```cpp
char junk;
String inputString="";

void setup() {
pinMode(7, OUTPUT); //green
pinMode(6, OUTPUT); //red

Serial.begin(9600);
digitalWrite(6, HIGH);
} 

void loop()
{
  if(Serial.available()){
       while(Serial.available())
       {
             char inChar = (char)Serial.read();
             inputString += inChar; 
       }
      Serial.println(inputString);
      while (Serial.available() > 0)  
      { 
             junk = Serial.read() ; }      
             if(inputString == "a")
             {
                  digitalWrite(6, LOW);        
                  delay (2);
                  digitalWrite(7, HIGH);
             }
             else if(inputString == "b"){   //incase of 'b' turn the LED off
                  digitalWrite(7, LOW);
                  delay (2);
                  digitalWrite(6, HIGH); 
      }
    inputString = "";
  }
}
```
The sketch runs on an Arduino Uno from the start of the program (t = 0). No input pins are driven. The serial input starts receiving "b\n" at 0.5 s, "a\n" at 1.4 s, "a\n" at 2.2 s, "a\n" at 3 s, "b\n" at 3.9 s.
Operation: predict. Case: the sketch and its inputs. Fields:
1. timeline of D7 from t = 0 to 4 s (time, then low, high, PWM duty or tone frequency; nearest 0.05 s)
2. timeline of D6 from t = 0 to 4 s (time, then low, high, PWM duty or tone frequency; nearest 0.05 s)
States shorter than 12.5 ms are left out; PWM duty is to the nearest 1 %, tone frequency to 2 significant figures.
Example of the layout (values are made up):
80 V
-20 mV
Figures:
0 s low; 1.4 s high; 3.9 s low
0 s high; 1.4 s low; 3.9 s high
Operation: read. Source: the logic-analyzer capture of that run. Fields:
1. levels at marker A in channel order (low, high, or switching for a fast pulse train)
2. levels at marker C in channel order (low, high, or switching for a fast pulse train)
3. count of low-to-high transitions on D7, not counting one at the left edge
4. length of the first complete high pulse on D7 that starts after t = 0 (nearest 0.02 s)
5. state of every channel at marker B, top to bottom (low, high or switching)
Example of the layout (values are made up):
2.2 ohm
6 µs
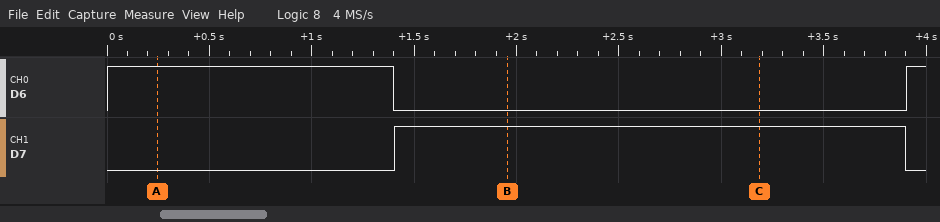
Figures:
D6 high, D7 low
D6 low, D7 high
1
2.50 s
D6 low, D7 high
